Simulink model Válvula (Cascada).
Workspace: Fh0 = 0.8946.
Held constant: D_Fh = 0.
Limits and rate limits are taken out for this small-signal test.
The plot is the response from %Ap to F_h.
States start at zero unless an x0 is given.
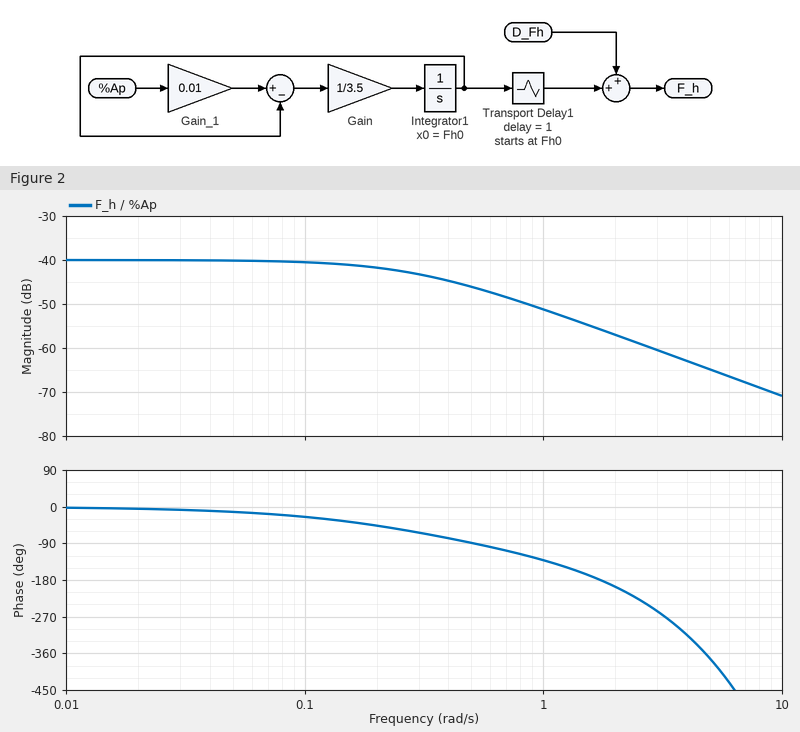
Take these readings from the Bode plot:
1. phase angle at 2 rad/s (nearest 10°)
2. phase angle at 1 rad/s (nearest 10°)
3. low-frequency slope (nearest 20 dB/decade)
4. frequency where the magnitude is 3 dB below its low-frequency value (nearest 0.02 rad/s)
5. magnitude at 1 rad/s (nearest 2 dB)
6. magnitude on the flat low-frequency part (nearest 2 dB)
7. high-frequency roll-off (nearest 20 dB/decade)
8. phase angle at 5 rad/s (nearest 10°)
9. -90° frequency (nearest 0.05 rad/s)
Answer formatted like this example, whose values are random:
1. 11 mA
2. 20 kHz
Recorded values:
1. -200°
2. -130°
3. 0 dB/decade
4. 0.28 rad/s
5. -52 dB
6. -40 dB
7. -20 dB/decade
8. -370°
9. 0.50 rad/s
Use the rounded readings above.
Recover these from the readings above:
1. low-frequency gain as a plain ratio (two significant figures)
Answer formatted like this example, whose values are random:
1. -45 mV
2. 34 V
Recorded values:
1. 0.010
